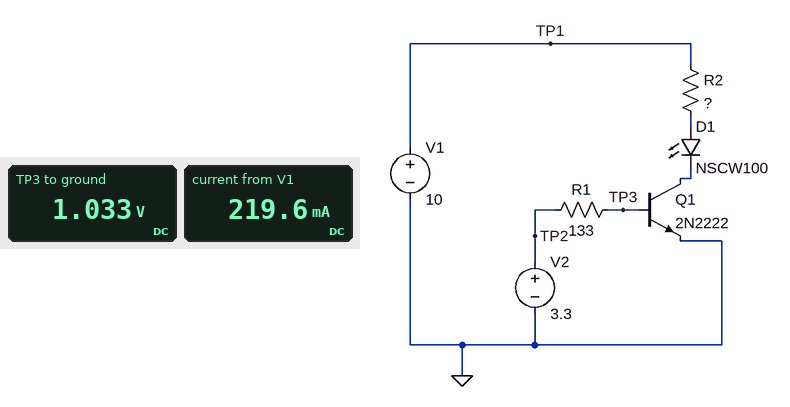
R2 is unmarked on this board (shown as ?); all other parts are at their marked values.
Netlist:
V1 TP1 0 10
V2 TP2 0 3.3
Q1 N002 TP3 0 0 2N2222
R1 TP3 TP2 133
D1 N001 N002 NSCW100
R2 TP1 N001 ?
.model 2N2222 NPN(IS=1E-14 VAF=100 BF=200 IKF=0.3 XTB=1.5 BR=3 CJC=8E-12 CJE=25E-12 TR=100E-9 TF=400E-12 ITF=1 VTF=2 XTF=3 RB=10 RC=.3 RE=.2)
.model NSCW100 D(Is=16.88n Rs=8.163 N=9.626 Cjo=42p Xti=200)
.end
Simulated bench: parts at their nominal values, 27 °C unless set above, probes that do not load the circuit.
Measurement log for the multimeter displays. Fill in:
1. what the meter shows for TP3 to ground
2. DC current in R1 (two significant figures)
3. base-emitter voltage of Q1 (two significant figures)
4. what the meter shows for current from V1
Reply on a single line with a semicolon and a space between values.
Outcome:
1.033 V; 17 mA; 1.0 V; 219.6 mA
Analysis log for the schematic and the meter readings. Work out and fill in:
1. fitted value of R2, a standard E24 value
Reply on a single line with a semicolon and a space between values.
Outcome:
18 Ω
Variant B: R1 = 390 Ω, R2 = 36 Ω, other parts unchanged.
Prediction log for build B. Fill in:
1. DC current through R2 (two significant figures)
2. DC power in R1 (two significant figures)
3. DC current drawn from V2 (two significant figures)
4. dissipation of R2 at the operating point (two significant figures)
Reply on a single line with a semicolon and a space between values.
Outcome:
130 mA; 15 mW; 6.2 mA; 640 mW
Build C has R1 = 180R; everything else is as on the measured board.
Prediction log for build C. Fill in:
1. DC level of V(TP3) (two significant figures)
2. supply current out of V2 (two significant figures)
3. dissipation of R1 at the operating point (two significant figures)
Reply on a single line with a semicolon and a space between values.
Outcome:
990 mV; 13 mA; 30 mW
